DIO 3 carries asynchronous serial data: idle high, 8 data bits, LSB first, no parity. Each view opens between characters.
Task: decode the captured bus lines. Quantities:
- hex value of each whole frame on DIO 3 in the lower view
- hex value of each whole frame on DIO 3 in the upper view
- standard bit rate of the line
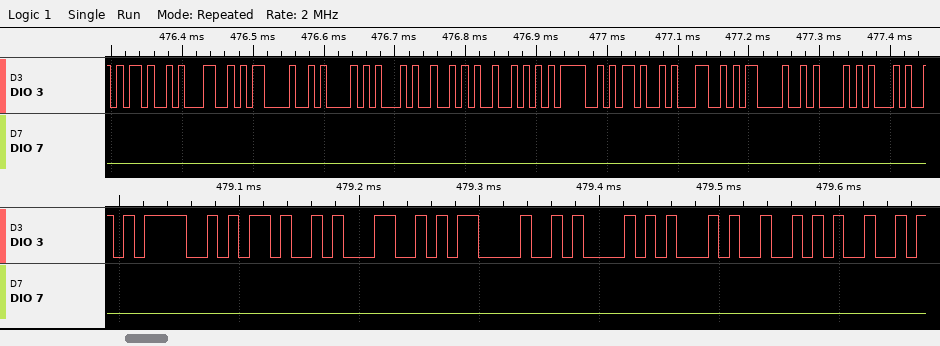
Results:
3D, 2D, 31, 0D, 0A, 45, 52
2D, 31, 0D, 0A, 45, 52, 52, 3D, 2D, 31, 0D, 0A, 45
115200 baud
